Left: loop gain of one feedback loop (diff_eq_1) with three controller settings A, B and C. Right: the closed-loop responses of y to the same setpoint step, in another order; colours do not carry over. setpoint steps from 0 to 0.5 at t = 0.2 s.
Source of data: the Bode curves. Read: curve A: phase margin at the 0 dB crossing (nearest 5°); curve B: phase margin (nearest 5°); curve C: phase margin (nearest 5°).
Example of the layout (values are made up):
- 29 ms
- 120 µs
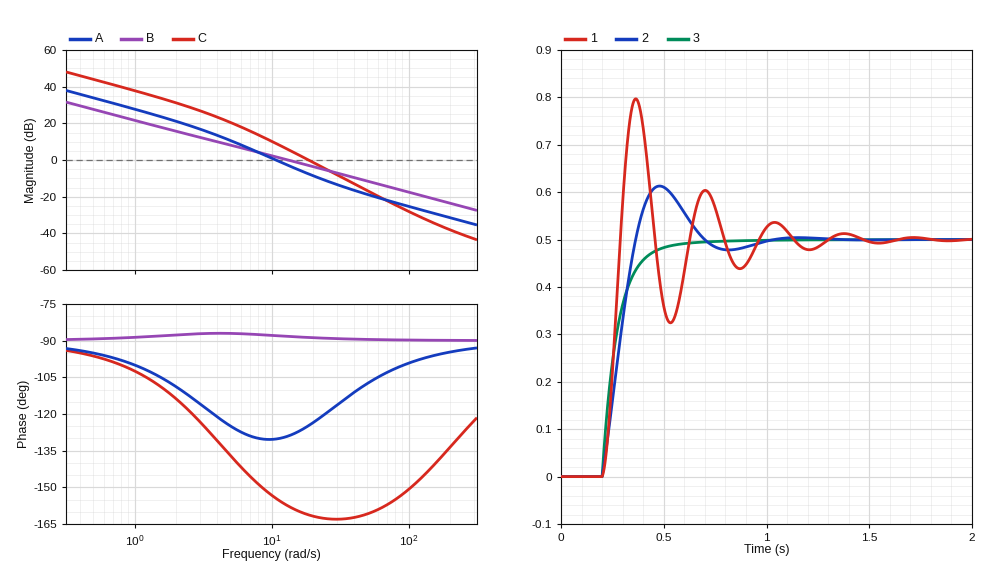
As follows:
- 50°
- 90°
- 20°
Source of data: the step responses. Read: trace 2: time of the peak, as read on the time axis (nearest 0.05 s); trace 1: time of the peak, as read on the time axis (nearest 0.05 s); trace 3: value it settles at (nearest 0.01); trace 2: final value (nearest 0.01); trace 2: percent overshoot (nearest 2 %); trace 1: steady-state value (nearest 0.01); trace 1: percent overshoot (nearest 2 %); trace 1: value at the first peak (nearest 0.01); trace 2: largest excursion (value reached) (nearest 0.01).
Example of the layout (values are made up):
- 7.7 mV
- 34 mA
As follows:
- 0.50 s
- 0.35 s
- 0.50
- 0.50
- 22 %
- 0.50
- 60 %
- 0.80
- 0.61
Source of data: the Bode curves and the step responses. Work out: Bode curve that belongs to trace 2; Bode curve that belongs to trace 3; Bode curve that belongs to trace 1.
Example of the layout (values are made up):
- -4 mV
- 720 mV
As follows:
- A
- B
- C
